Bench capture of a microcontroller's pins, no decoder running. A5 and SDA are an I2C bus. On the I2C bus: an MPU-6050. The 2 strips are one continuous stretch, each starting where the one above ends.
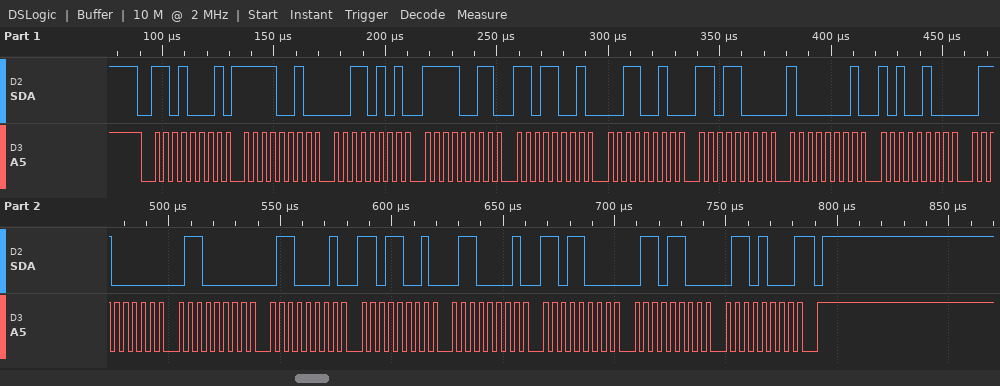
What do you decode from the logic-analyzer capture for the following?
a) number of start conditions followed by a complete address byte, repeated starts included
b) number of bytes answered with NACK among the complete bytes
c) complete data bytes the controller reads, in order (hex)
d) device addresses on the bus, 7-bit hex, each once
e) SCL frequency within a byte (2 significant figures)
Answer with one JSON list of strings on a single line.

["1", "1", "F2 35 F3 D9 32 D8 81 A4 60 60 61 D9 61 D8 6C 68", "0x68", "250 kHz"]
